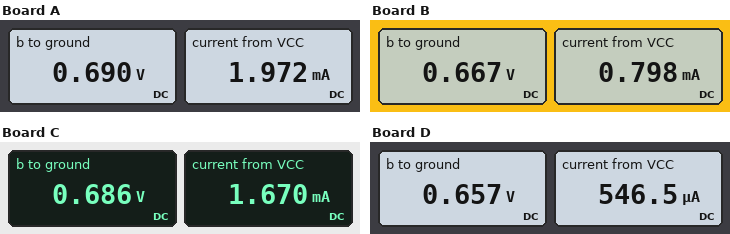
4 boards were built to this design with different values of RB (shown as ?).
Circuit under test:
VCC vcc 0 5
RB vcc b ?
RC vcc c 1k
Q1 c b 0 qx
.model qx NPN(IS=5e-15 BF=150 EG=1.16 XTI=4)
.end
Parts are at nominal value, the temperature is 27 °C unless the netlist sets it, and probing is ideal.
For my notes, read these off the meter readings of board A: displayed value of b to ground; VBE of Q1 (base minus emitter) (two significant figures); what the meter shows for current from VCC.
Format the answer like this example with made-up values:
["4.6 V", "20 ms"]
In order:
["0.690 V", "690 mV", "1.972 mA"]
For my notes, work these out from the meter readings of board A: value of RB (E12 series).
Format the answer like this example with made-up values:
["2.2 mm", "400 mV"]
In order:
["330 kΩ"]
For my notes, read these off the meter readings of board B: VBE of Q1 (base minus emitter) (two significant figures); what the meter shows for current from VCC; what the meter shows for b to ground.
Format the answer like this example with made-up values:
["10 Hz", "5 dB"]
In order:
["670 mV", "0.798 mA", "0.667 V"]
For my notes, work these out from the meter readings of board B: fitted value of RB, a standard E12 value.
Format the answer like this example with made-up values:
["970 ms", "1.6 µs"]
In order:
["820 kΩ"]
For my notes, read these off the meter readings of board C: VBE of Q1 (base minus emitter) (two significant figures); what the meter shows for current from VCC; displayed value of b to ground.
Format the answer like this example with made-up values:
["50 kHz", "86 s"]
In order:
["690 mV", "1.670 mA", "0.686 V"]
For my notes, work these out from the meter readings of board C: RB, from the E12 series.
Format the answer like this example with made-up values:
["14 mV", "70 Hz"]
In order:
["390 kΩ"]
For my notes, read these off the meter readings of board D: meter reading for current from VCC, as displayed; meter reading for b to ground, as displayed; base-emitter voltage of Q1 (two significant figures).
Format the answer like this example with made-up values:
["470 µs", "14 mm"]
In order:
["546.5 µA", "0.657 V", "660 mV"]
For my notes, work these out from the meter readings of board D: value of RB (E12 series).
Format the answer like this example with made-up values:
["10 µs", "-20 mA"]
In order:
["1.2 MΩ"]
